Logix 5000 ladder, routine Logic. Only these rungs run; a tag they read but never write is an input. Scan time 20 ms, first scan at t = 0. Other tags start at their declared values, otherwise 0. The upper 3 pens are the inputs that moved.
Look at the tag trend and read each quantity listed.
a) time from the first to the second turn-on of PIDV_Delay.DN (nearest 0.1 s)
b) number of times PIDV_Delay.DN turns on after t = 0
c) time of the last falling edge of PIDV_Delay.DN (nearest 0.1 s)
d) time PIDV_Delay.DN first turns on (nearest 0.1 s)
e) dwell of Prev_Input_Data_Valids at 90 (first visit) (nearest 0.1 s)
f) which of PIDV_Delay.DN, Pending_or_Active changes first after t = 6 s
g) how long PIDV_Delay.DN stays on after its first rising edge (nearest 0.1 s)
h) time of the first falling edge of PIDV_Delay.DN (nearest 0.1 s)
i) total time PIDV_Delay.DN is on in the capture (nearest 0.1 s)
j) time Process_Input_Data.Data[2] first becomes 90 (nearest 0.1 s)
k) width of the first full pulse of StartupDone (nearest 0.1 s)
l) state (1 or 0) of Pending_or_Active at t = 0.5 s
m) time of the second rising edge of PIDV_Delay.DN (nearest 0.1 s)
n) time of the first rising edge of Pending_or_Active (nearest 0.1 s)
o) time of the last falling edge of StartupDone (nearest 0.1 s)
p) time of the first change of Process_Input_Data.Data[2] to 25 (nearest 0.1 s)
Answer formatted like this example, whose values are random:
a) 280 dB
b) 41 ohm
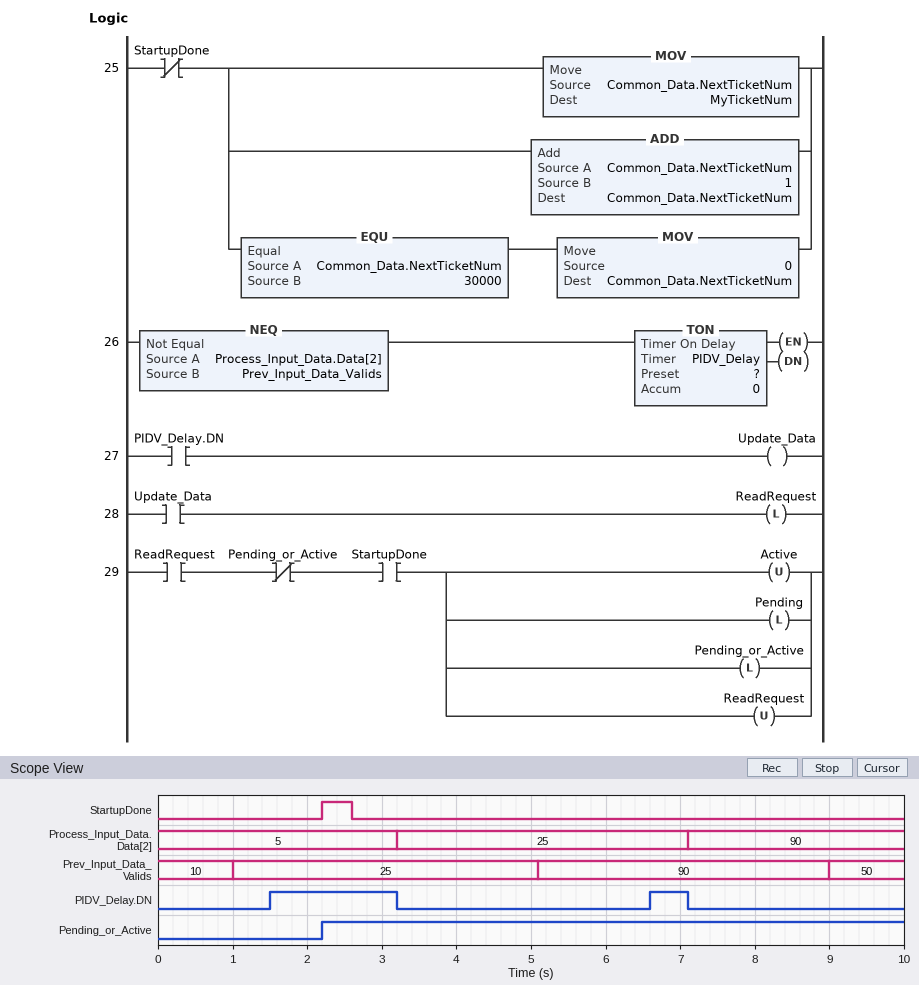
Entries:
a) 5.1 s
b) 2
c) 7.1 s
d) 1.5 s
e) 3.9 s
f) PIDV_Delay.DN
g) 1.7 s
h) 3.2 s
i) 2.2 s
j) 7.1 s
k) 0.4 s
l) 0
m) 6.6 s
n) 2.2 s
o) 2.6 s
p) 3.2 s
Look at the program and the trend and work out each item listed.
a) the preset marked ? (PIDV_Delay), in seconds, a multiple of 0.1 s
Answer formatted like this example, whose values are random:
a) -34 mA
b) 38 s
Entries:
a) 1.5 s
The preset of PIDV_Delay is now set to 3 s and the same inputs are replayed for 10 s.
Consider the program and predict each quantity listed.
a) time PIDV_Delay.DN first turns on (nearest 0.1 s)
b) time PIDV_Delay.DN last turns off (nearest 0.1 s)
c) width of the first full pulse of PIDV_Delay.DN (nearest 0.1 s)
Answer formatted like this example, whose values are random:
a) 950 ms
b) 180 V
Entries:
a) 3.0 s
b) 3.2 s
c) 0.2 s
